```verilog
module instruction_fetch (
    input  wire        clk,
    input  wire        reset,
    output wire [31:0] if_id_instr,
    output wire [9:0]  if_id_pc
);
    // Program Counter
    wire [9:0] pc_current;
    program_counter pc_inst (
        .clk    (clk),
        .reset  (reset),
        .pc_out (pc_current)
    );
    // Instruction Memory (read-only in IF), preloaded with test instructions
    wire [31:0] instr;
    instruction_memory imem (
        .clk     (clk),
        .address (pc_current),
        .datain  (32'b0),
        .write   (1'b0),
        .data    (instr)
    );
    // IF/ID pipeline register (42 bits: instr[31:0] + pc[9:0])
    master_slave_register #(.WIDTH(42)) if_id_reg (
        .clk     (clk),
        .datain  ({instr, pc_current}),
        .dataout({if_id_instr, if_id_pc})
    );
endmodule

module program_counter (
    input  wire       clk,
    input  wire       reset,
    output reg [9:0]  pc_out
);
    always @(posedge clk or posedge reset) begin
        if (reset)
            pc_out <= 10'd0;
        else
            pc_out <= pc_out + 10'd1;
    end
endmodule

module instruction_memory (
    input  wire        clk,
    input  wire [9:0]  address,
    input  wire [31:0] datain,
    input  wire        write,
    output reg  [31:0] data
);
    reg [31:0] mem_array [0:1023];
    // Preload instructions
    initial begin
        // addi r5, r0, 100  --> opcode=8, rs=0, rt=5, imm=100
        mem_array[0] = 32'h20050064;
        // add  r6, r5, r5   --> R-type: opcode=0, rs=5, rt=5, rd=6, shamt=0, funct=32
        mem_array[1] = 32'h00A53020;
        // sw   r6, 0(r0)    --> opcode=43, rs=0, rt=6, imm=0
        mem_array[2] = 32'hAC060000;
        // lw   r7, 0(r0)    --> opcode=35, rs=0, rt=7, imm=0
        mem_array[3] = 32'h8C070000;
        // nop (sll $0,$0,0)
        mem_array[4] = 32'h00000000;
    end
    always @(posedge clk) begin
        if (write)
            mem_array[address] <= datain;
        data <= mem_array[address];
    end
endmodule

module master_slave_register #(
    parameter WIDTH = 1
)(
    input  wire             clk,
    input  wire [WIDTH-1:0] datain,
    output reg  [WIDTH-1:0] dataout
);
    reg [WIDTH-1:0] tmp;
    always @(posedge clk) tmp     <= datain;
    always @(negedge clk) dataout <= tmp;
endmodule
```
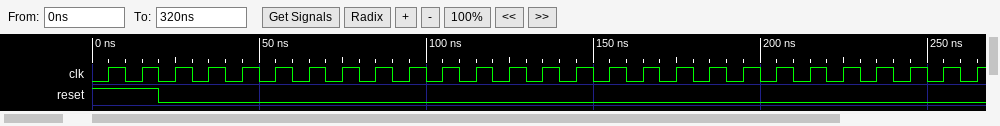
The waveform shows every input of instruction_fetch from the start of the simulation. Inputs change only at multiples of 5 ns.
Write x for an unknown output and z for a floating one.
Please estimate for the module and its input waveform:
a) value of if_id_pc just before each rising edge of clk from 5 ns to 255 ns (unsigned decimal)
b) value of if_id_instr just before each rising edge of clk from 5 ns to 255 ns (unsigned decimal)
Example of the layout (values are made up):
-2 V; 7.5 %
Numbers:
x, 0, 0, 0, 1, 2, 3, 4, 5, 6, 7, 8, 9, 10, 11, 12, 13, 14, 15, 16, 17, 18, 19, 20, 21, 22; x, x, 537198692, 537198692, 537198692, 10825760, 2886074368, 2349268992, 0, x, x, x, x, x, x, x, x, x, x, x, x, x, x, x, x, x
